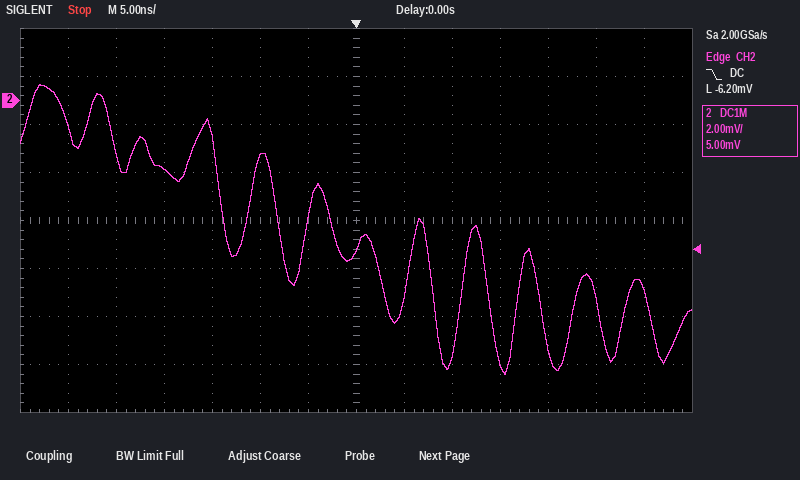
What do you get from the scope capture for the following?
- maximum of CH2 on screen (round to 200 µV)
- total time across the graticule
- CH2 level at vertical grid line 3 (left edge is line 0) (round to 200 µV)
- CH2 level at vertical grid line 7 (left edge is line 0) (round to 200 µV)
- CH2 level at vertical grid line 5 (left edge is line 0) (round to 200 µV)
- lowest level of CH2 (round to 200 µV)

600 µV
70 ns
-2.8 mV
-6.2 mV
-2.4 mV
-11.4 mV
